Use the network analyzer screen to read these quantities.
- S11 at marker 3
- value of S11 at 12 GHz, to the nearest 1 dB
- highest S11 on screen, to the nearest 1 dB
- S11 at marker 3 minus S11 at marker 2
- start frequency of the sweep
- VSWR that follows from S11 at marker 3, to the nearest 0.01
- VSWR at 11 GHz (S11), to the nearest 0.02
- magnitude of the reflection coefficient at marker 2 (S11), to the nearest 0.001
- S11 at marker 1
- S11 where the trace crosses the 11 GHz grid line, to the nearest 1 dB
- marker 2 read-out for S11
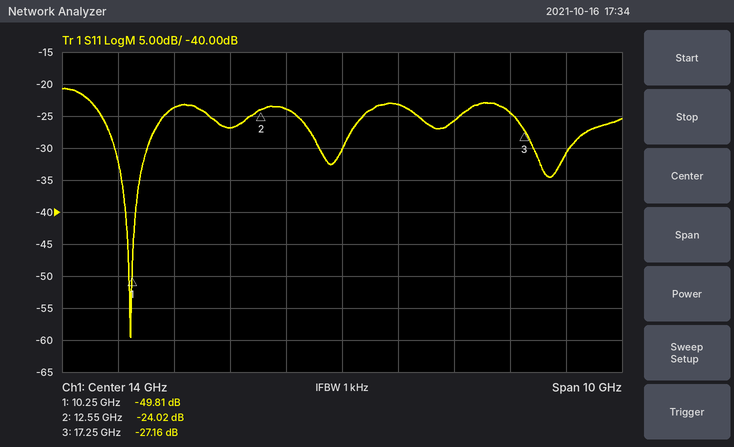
-27.16 dB
-27 dB
-21 dB
-3.14 dB
9 GHz
1.09
1.14
0.063
-49.81 dB
-24 dB
-24.02 dB
